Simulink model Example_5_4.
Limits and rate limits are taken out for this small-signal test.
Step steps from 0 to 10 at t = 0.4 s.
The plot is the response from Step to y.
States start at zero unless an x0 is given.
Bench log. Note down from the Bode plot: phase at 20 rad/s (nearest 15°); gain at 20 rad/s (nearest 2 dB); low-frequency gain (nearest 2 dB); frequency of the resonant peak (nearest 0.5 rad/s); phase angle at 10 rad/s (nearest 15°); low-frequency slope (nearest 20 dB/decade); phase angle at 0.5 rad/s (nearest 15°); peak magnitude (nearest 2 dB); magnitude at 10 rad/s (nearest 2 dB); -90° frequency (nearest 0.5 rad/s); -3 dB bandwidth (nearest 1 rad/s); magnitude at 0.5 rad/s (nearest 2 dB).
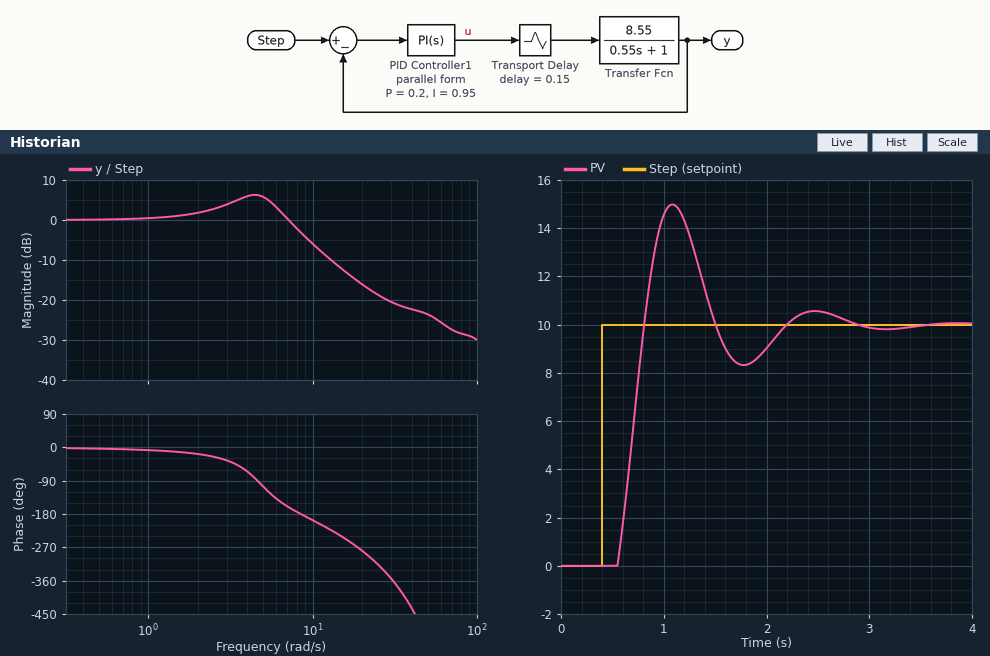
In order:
-285°
-16 dB
0 dB
4.5 rad/s
-195°
0 dB/decade
0°
6 dB
-6 dB
4.5 rad/s
8 rad/s
0 dB
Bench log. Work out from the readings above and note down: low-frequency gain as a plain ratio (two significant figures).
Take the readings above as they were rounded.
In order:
1.0
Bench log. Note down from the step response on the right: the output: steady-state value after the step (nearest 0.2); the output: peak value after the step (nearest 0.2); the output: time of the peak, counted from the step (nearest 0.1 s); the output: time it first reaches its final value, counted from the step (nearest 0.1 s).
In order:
10.0
15.0
0.7 s
0.4 s
